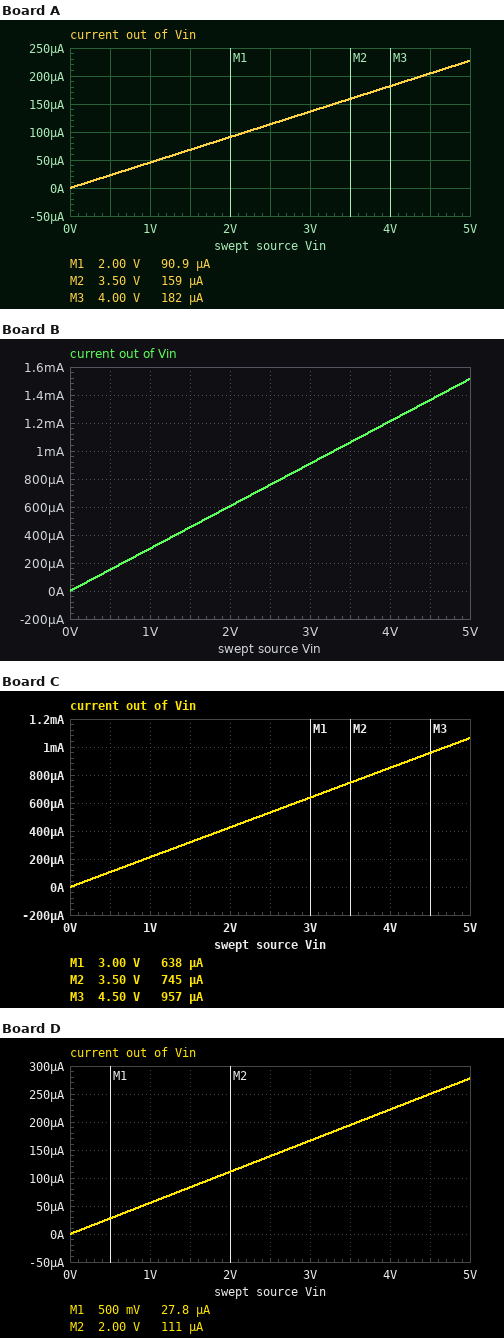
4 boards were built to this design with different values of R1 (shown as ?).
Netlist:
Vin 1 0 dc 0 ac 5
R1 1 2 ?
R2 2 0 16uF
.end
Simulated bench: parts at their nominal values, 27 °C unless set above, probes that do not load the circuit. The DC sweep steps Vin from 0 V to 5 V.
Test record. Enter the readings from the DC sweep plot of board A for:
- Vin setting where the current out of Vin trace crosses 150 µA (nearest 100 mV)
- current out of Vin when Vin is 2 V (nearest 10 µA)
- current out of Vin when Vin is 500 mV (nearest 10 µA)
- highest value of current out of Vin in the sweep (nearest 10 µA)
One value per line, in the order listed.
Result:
3.3 V
90 µA
20 µA
230 µA
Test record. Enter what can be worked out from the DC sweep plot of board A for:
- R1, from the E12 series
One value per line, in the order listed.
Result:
22 kΩ
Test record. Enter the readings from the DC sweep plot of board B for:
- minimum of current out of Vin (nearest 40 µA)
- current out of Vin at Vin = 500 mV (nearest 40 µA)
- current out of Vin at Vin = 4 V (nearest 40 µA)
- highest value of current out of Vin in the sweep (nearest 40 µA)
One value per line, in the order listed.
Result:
0 A
160 µA
1.20 mA
1.52 mA
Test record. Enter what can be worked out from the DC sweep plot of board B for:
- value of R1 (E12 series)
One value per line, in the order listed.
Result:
3.3 kΩ
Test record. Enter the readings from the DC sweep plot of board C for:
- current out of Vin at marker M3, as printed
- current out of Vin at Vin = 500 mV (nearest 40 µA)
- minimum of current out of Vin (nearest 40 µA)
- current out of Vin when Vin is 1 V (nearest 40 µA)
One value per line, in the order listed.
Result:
957 µA
120 µA
0 A
200 µA
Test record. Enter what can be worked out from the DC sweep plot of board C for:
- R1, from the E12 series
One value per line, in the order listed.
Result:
4.7 kΩ
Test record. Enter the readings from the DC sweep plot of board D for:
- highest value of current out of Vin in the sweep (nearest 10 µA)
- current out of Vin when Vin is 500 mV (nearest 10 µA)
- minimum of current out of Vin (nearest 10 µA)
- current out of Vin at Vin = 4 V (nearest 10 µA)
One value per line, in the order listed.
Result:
280 µA
30 µA
0 A
220 µA
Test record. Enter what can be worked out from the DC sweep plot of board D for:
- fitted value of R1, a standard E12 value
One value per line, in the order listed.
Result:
18 kΩ
